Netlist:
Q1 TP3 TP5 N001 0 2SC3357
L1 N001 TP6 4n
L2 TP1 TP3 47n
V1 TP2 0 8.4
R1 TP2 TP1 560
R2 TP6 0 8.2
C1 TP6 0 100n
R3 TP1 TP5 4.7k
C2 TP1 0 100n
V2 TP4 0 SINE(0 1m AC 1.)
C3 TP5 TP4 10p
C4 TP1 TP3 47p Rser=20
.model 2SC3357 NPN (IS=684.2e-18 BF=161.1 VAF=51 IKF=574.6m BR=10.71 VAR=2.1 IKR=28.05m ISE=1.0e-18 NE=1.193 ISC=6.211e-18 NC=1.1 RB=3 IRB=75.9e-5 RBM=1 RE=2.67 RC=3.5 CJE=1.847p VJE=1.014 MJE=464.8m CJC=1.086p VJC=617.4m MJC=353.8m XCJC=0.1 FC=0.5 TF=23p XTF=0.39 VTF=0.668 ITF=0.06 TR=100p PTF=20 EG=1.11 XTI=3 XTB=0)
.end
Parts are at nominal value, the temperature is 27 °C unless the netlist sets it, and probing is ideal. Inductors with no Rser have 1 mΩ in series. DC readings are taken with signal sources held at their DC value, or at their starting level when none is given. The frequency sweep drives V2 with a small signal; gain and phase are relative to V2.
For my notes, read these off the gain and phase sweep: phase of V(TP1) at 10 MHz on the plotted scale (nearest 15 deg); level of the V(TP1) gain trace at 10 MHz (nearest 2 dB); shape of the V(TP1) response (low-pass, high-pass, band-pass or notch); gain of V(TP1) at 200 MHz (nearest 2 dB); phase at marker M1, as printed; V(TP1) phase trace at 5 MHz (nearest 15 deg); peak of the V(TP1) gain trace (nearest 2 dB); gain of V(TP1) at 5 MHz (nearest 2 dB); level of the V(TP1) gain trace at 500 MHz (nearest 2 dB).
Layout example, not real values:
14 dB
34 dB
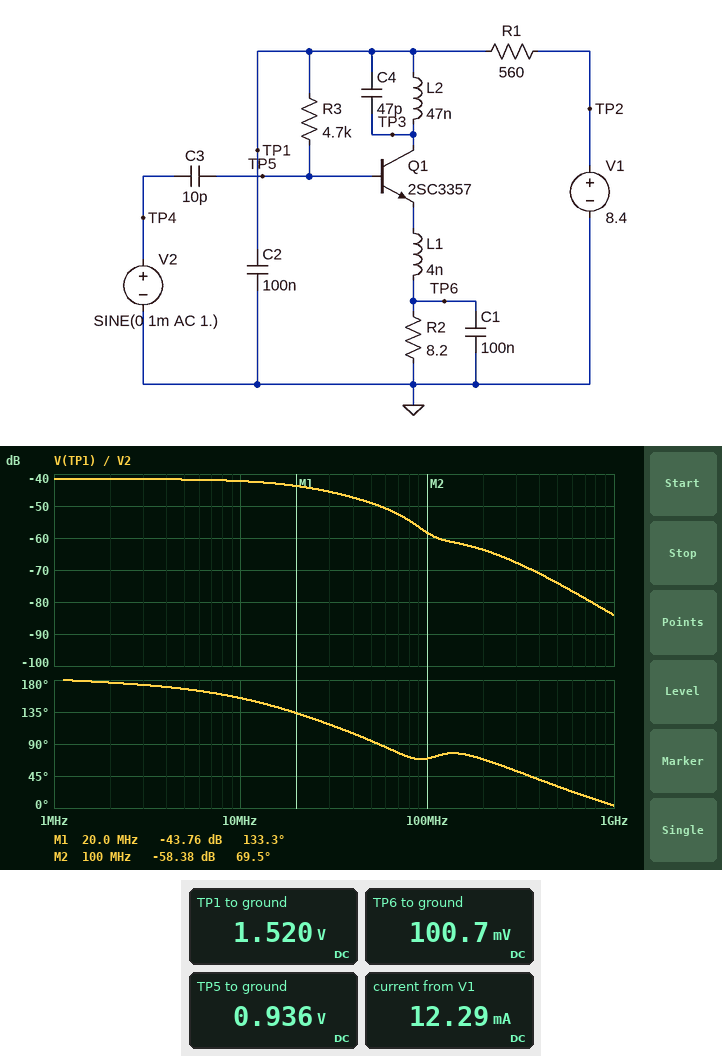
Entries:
150 deg
-42 dB
low-pass
-64 dB
133.3 deg
165 deg
-42 dB
-42 dB
-74 dB
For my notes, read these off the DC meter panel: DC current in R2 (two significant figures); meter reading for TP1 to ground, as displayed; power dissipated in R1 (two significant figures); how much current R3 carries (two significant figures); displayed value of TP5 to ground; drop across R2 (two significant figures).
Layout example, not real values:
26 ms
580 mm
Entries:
12 mA
1.520 V
85 mW
120 µA
0.936 V
100 mV
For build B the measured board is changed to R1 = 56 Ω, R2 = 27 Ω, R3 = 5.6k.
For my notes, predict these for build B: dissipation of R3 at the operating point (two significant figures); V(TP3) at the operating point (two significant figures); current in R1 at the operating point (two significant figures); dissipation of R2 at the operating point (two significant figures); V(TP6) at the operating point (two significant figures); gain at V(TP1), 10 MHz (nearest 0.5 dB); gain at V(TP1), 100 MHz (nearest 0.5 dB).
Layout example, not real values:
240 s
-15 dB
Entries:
1.7 mW
5.5 V
52 mA
73 mW
1.4 V
-42.5 dB
-55.5 dB
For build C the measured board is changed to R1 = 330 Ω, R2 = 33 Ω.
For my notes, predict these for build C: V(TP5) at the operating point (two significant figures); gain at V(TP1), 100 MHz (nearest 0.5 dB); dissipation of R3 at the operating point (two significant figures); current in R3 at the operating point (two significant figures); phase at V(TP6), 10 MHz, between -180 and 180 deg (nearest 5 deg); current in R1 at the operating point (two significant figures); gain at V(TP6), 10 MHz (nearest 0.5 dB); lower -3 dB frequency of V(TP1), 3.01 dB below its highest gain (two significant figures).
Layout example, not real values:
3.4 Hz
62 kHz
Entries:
1.5 V
-57.5 dB
170 µW
190 µA
-20 deg
18 mA
-42.0 dB
69 kHz
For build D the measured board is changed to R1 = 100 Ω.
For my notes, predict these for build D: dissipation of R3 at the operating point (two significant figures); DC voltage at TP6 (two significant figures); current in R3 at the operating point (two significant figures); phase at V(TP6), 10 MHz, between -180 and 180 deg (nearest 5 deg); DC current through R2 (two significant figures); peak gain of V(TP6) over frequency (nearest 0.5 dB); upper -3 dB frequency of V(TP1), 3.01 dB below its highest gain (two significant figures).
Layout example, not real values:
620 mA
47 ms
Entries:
1.2 mW
380 mV
500 µA
-15 deg
47 mA
-42.5 dB
41 MHz
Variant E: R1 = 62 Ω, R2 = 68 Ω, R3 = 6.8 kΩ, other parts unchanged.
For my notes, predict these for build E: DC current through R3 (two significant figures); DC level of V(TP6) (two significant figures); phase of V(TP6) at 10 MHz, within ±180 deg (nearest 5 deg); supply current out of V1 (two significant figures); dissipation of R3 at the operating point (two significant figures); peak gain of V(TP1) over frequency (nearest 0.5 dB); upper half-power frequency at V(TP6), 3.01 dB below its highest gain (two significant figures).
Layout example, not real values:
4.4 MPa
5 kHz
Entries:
390 µA
2.5 V
-20 deg
37 mA
1.0 mW
-42.0 dB
37 MHz
